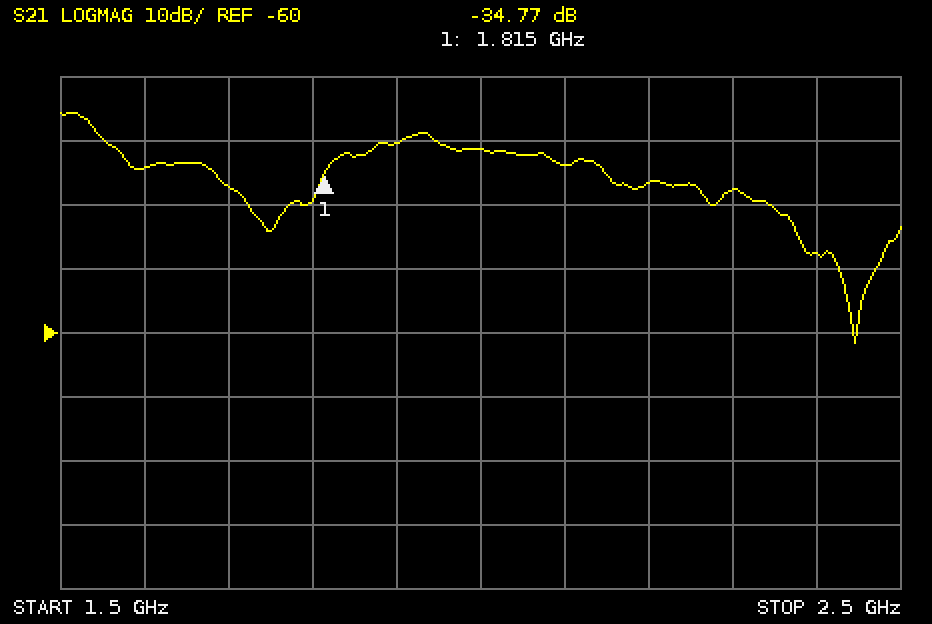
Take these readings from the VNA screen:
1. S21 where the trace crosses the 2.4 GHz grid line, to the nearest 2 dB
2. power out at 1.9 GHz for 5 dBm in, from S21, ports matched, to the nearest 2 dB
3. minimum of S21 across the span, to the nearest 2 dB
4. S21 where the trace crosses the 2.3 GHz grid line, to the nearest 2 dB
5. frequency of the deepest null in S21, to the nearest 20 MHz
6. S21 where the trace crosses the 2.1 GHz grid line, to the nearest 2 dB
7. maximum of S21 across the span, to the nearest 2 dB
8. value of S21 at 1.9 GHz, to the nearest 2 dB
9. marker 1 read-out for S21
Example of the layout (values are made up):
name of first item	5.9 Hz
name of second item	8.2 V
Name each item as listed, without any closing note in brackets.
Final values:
S21 where the trace crosses the 2.4 GHz grid line, to the nearest 2 dB	-48 dB
power out at 1.9 GHz for 5 dBm in, from S21, ports matched, to the nearest 2 dB	-26 dBm
minimum of S21 across the span, to the nearest 2 dB	-62 dB
S21 where the trace crosses the 2.3 GHz grid line, to the nearest 2 dB	-38 dB
frequency of the deepest null in S21, to the nearest 20 MHz	2.44 GHz
S21 where the trace crosses the 2.1 GHz grid line, to the nearest 2 dB	-34 dB
maximum of S21 across the span, to the nearest 2 dB	-26 dB
value of S21 at 1.9 GHz, to the nearest 2 dB	-30 dB
marker 1 read-out for S21	-34.77 dB
